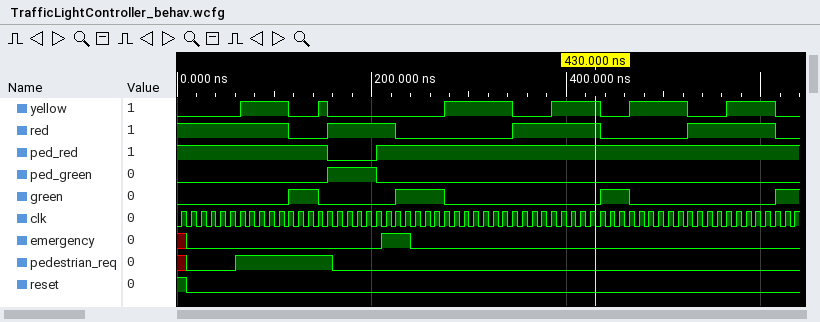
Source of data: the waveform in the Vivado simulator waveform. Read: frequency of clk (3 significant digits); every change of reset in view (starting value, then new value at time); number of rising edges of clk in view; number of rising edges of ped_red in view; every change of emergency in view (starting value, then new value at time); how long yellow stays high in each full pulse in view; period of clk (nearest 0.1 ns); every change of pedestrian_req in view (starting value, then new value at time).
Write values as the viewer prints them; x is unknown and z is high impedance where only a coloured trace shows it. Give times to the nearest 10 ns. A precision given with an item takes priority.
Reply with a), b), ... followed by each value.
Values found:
a) 100 MHz
b) 1, 0 at 10 ns
c) 64
d) 1
e) x, 0 at 10 ns, 1 at 210 ns, 0 at 240 ns
f) 50 ns, 10 ns, 70 ns, 50 ns, 60 ns, 50 ns
g) 10 ns
h) x, 0 at 10 ns, 1 at 60 ns, 0 at 160 ns
